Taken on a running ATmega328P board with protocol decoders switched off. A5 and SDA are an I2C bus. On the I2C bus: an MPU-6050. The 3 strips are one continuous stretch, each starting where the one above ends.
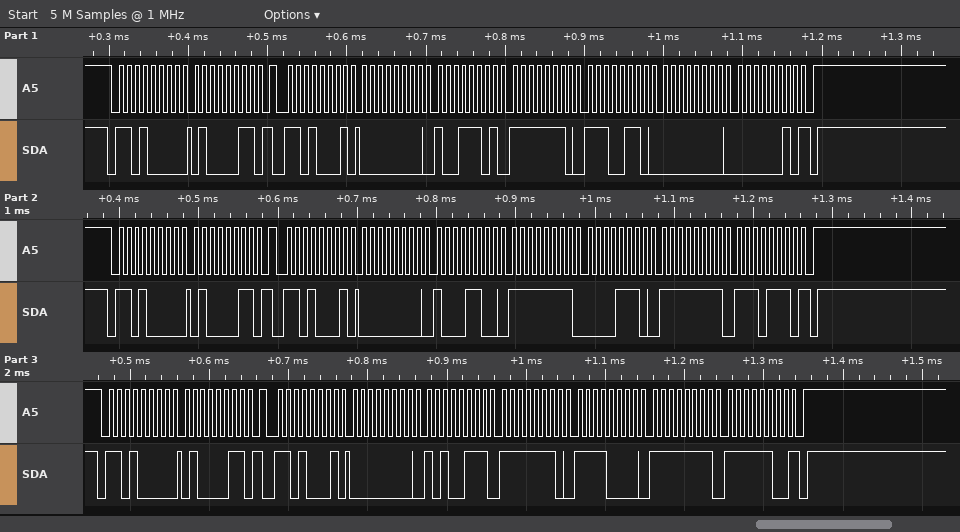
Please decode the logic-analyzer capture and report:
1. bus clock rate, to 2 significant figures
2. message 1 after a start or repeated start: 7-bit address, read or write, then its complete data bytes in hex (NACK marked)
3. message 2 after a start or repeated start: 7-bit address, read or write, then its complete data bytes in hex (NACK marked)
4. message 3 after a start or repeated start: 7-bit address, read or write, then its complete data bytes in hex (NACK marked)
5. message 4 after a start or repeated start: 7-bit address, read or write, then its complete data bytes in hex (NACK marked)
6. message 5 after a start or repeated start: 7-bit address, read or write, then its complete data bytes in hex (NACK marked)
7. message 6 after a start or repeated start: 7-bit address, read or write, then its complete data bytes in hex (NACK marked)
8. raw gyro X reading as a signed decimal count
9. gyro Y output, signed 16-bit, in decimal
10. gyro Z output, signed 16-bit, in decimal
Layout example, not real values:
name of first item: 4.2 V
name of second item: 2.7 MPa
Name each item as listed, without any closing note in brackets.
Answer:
bus clock rate, to 2 significant figures: 100 kHz
message 1 after a start or repeated start: 7-bit address, read or write, then its complete data bytes in hex: 0x68 write: 43
message 2 after a start or repeated start: 7-bit address, read or write, then its complete data bytes in hex: 0x68 read: 00 9D FE E6 00 02 NACK
message 3 after a start or repeated start: 7-bit address, read or write, then its complete data bytes in hex: 0x68 write: 43
message 4 after a start or repeated start: 7-bit address, read or write, then its complete data bytes in hex: 0x68 read: 00 8C FF 0E FF EE NACK
message 5 after a start or repeated start: 7-bit address, read or write, then its complete data bytes in hex: 0x68 write: 43
message 6 after a start or repeated start: 7-bit address, read or write, then its complete data bytes in hex: 0x68 read: 00 A7 FE F0 FF FC NACK
raw gyro X reading as a signed decimal count: 157
gyro Y output, signed 16-bit, in decimal: -282
gyro Z output, signed 16-bit, in decimal: 2
